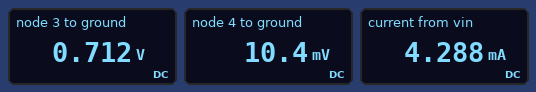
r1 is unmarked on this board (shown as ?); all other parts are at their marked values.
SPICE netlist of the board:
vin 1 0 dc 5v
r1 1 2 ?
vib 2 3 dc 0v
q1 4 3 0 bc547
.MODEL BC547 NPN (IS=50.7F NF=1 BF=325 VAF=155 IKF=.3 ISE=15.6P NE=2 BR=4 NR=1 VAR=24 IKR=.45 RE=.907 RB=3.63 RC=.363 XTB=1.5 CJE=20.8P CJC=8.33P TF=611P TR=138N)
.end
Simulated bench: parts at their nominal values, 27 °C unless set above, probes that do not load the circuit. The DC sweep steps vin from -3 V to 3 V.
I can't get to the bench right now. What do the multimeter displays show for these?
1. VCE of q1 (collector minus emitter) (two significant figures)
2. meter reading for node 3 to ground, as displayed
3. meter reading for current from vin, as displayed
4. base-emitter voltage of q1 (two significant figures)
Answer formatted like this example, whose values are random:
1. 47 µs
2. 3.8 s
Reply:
1. 10 mV
2. 0.712 V
3. 4.288 mA
4. 710 mV
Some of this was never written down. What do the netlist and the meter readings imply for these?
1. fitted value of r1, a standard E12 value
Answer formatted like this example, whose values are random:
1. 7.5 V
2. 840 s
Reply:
1. 1 kΩ
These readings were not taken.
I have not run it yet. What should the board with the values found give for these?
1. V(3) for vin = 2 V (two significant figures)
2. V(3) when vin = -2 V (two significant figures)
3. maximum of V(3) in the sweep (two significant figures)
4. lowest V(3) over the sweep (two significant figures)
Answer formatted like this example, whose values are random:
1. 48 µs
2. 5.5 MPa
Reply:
1. 670 mV
2. -2.0 V
3. 690 mV
4. -3.0 V
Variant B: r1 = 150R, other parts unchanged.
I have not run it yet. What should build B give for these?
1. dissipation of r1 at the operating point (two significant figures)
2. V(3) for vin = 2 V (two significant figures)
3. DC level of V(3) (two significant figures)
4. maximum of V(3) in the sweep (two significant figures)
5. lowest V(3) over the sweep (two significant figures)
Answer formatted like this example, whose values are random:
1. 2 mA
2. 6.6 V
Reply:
1. 110 mW
2. 750 mV
3. 870 mV
4. 790 mV
5. -3.0 V
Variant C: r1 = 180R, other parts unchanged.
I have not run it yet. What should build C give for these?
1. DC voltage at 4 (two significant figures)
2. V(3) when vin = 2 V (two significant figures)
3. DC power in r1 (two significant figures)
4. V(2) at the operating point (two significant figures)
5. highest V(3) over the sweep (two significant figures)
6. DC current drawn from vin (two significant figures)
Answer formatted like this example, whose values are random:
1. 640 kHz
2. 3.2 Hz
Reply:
1. 29 mV
2. 740 mV
3. 96 mW
4. 840 mV
5. 780 mV
6. 23 mA
